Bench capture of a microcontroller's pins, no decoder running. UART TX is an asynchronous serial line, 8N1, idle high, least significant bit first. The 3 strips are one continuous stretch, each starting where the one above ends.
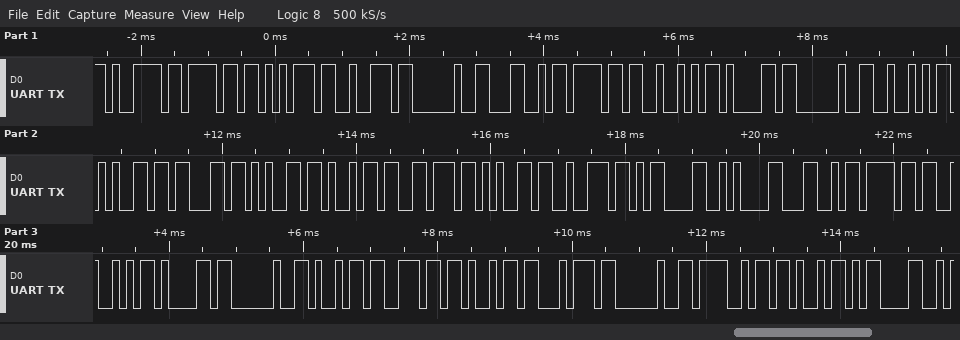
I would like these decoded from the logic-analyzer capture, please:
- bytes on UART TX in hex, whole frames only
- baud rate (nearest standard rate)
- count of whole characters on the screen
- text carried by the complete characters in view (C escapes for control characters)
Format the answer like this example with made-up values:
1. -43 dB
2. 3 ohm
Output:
1. 79 6F 75 72 20 4C 6F 52 61 20 52 65 63 65 69 76 65 72 0D 0A 4C 6F 52 61 20 69 6E 69 74 20 4F 4B 0D
2. 9600 baud
3. 33
4. "your LoRa Receiver\r\nLoRa init OK\r"
